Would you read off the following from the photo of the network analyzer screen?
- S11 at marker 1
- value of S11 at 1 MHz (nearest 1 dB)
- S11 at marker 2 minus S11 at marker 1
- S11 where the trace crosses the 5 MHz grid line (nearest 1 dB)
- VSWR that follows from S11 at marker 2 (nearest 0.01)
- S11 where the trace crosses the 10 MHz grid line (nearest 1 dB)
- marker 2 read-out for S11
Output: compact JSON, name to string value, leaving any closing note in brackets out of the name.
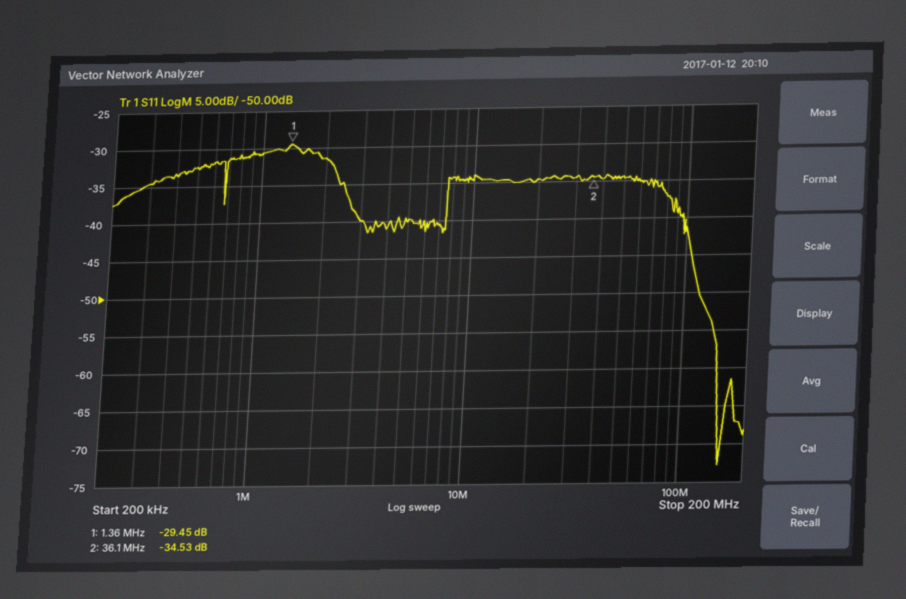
{"S11 at marker 1": "-29.45 dB", "value of S11 at 1 MHz": "-31 dB", "S11 at marker 2 minus S11 at marker 1": "-5.08 dB", "S11 where the trace crosses the 5 MHz grid line": "-40 dB", "VSWR that follows from S11 at marker 2": "1.04", "S11 where the trace crosses the 10 MHz grid line": "-34 dB", "marker 2 read-out for S11": "-34.53 dB"}
